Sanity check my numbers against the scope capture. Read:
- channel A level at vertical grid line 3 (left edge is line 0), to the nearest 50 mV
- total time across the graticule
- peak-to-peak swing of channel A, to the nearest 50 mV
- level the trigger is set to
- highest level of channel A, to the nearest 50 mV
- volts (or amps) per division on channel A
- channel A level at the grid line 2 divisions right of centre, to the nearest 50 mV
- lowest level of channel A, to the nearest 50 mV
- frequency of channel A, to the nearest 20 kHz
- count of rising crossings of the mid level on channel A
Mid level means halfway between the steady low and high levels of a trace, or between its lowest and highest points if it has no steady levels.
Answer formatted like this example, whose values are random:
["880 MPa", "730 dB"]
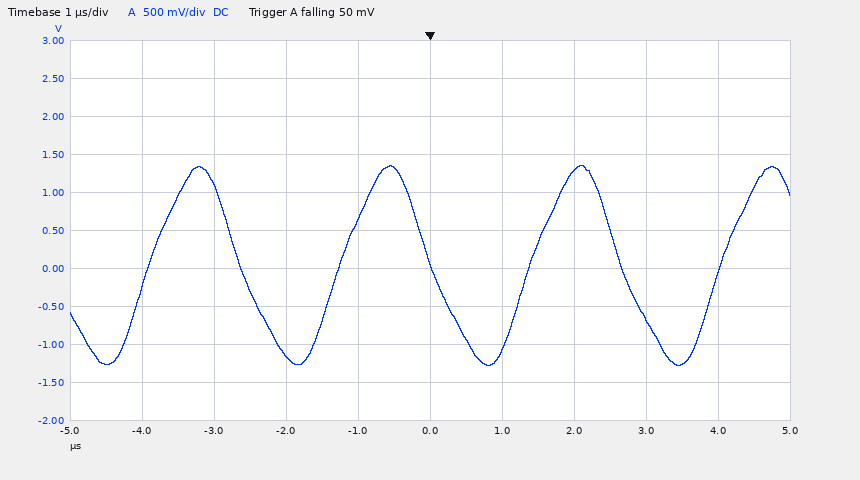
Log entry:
["-1.15 V", "10 µs", "2.65 V", "50 mV", "1.35 V", "500 mV", "1.30 V", "-1.30 V", "380 kHz", "4"]
